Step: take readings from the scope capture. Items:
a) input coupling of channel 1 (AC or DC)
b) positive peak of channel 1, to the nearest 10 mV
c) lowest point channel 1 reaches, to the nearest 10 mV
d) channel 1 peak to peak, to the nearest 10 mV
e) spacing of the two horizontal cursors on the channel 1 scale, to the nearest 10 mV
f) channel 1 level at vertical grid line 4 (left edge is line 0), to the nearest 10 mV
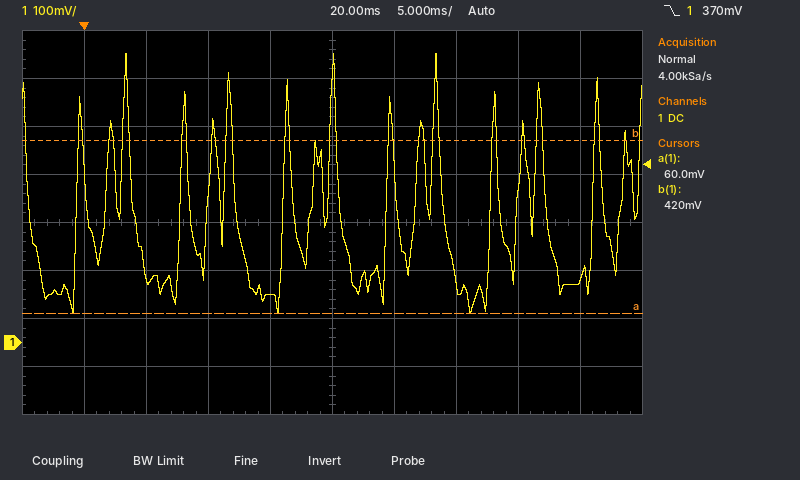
DC
600 mV
60 mV
540 mV
360 mV
100 mV
